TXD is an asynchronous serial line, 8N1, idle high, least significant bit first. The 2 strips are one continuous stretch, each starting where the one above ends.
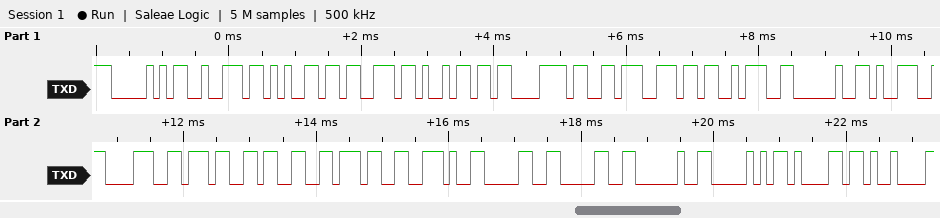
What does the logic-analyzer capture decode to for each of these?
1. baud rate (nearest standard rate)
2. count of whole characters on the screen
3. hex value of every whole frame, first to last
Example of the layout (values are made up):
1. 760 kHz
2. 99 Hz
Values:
1. 9600 baud
2. 22
3. 50 72 65 73 69 C3 B3 6E 3A 20 39 38 37 33 37 2E 30 30 20 50 61 09
